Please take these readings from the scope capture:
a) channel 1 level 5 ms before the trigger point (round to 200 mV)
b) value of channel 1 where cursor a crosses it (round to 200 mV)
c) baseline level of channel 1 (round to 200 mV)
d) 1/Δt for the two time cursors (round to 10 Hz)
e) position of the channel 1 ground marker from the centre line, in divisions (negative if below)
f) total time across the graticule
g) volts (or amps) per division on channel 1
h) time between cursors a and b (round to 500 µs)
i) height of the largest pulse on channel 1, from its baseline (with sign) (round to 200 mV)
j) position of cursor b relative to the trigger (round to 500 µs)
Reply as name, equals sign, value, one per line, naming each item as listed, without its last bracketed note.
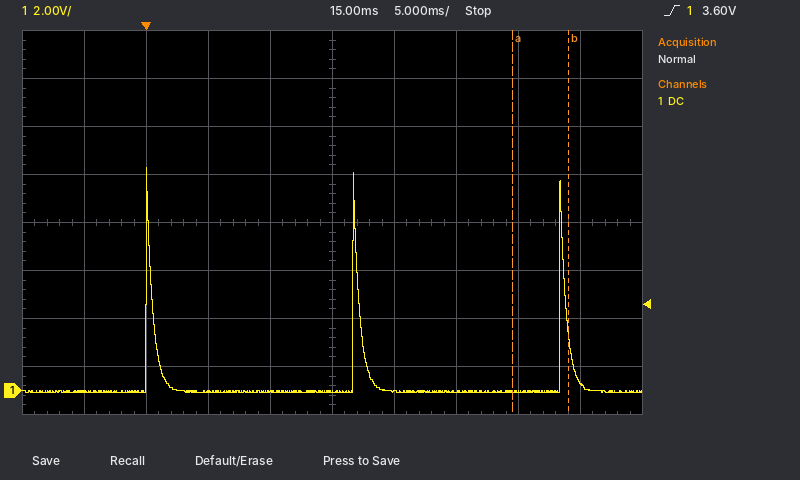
channel 1 level 5 ms before the trigger point = 0.0 V
value of channel 1 where cursor a crosses it = 0.0 V
baseline level of channel 1 = 0.0 V
1/Δt for the two time cursors = 220 Hz
position of the channel 1 ground marker from the centre line, in divisions = -3.5 div
total time across the graticule = 50 ms
volts (or amps) per division on channel 1 = 2 V
time between cursors a and b = 4.5 ms
height of the largest pulse on channel 1, from its baseline (with sign) = +9.4 V
position of cursor b relative to the trigger = +34.0 ms
